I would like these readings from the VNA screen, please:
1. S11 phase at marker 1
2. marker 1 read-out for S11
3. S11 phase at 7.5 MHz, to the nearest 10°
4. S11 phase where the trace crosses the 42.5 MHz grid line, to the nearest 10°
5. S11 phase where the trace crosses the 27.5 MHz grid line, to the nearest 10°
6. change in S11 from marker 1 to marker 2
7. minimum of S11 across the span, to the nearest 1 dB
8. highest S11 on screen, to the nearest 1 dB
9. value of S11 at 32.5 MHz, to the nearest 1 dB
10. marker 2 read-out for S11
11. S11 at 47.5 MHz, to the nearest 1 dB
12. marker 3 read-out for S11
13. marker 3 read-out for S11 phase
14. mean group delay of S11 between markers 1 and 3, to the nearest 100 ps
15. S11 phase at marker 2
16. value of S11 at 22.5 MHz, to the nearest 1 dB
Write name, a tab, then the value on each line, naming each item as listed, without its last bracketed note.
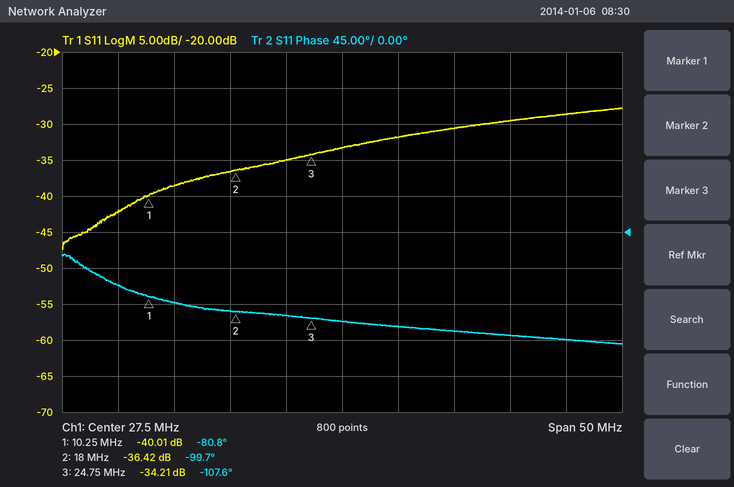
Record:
S11 phase at marker 1	-80.8°
marker 1 read-out for S11	-40.01 dB
S11 phase at 7.5 MHz, to the nearest 10°	-70°
S11 phase where the trace crosses the 42.5 MHz grid line, to the nearest 10°	-130°
S11 phase where the trace crosses the 27.5 MHz grid line, to the nearest 10°	-110°
change in S11 from marker 1 to marker 2	3.59 dB
minimum of S11 across the span, to the nearest 1 dB	-47 dB
highest S11 on screen, to the nearest 1 dB	-28 dB
value of S11 at 32.5 MHz, to the nearest 1 dB	-32 dB
marker 2 read-out for S11	-36.42 dB
S11 at 47.5 MHz, to the nearest 1 dB	-29 dB
marker 3 read-out for S11	-34.21 dB
marker 3 read-out for S11 phase	-107.6°
mean group delay of S11 between markers 1 and 3, to the nearest 100 ps	5.1 ns
S11 phase at marker 2	-99.7°
value of S11 at 22.5 MHz, to the nearest 1 dB	-35 dB
